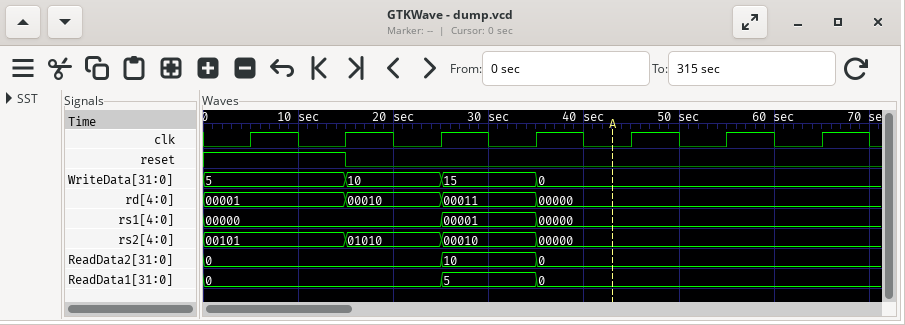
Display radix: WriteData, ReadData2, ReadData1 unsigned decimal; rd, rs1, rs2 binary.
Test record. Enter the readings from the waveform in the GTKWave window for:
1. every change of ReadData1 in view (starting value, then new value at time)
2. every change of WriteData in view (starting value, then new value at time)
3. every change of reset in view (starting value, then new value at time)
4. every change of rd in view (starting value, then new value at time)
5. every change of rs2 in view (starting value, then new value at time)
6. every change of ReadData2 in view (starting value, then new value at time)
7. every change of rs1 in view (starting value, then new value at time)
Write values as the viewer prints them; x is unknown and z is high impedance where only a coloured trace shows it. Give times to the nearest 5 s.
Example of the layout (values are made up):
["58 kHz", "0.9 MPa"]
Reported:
["0, 5 at 25 s, 0 at 35 s", "5, 10 at 15 s, 15 at 25 s, 0 at 35 s", "1, 0 at 15 s", "00001, 00010 at 15 s, 00011 at 25 s, 00000 at 35 s", "00101, 01010 at 15 s, 00010 at 25 s, 00000 at 35 s", "0, 10 at 25 s, 0 at 35 s", "00000, 00001 at 25 s, 00000 at 35 s"]
